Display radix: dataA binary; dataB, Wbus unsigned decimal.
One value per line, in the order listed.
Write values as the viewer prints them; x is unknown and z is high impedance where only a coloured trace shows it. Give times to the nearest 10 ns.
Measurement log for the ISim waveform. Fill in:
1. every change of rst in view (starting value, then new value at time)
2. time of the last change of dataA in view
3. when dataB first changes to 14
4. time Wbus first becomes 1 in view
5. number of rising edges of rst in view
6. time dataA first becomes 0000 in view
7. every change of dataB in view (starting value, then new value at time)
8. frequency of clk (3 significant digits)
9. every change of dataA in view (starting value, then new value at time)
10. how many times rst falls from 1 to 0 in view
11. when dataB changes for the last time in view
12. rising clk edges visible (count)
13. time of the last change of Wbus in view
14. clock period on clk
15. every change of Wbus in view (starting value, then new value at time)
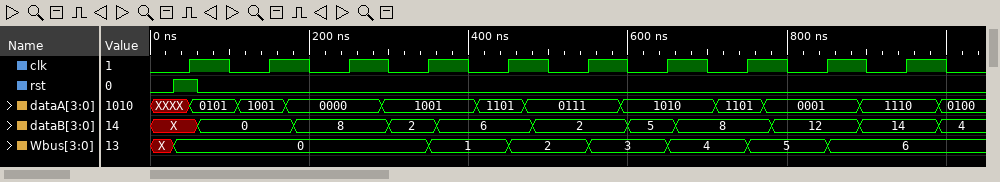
0, 1 at 30 ns, 0 at 60 ns
990 ns
890 ns
350 ns
1
170 ns
X, 0 at 60 ns, 8 at 180 ns, 2 at 300 ns, 6 at 360 ns, 2 at 480 ns, 5 at 600 ns, 8 at 660 ns, 12 at 780 ns, 14 at 890 ns, 4 at 990 ns
10.0 MHz
XXXX, 0101 at 50 ns, 1001 at 110 ns, 0000 at 170 ns, 1001 at 290 ns, 1101 at 410 ns, 0111 at 470 ns, 1010 at 590 ns, 1101 at 710 ns, 0001 at 770 ns, 1110 at 890 ns, 0100 at 990 ns
1
990 ns
10
850 ns
100 ns
X, 0 at 30 ns, 1 at 350 ns, 2 at 450 ns, 3 at 550 ns, 4 at 650 ns, 5 at 750 ns, 6 at 850 ns
